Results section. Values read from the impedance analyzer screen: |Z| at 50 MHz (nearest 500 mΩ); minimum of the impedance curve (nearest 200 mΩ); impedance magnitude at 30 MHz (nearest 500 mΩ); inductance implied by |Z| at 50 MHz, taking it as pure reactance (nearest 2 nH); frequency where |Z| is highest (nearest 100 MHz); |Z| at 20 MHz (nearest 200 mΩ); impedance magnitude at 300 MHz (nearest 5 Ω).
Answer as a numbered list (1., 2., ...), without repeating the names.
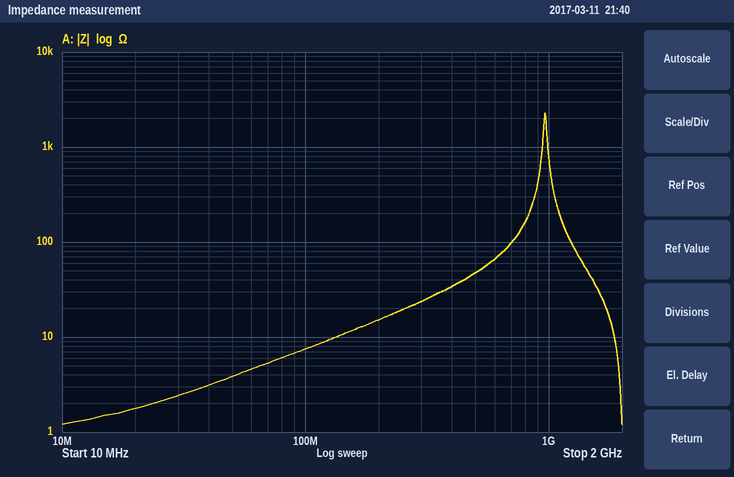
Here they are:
1. 4.0 Ω
2. 1.2 Ω
3. 2.5 Ω
4. 12 nH
5. 1.0 GHz
6. 1.8 Ω
7. 25 Ω
